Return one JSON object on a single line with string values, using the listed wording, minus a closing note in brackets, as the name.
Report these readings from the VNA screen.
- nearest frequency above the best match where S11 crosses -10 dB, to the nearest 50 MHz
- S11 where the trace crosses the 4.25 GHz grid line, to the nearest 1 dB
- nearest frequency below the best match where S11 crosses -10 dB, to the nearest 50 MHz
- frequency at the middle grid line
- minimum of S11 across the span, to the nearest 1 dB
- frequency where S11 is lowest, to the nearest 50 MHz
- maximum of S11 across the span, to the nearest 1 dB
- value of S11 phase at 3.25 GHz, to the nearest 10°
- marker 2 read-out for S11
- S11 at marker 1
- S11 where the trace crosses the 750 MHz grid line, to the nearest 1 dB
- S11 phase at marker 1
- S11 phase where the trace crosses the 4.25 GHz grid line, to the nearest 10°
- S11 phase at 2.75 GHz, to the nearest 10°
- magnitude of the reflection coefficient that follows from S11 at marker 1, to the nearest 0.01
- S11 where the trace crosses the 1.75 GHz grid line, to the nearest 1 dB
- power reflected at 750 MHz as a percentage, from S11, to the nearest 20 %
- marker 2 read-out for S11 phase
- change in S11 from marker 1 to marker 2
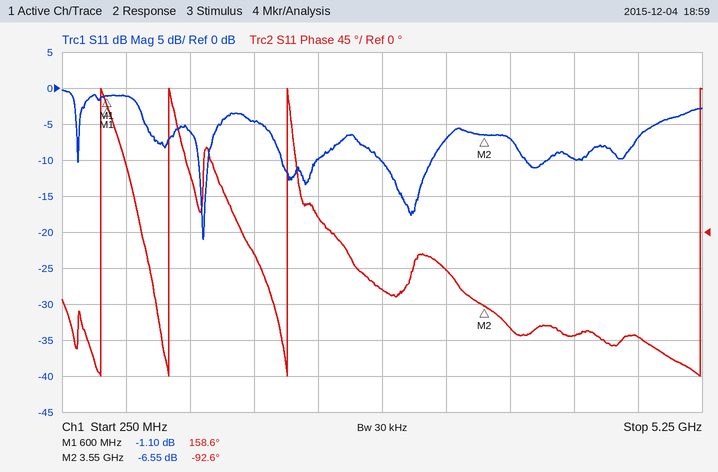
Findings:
{"nearest frequency above the best match where S11 crosses -10 dB, to the nearest 50 MHz": "1.40 GHz", "S11 where the trace crosses the 4.25 GHz grid line, to the nearest 1 dB": "-10 dB", "nearest frequency below the best match where S11 crosses -10 dB, to the nearest 50 MHz": "1.30 GHz", "frequency at the middle grid line": "2.75 GHz", "minimum of S11 across the span, to the nearest 1 dB": "-21 dB", "frequency where S11 is lowest, to the nearest 50 MHz": "1.35 GHz", "maximum of S11 across the span, to the nearest 1 dB": "0 dB", "value of S11 phase at 3.25 GHz, to the nearest 10°": "-50°", "marker 2 read-out for S11": "-6.55 dB", "S11 at marker 1": "-1.10 dB", "S11 where the trace crosses the 750 MHz grid line, to the nearest 1 dB": "-1 dB", "S11 phase at marker 1": "158.6°", "S11 phase where the trace crosses the 4.25 GHz grid line, to the nearest 10°": "-130°", "S11 phase at 2.75 GHz, to the nearest 10°": "-70°", "magnitude of the reflection coefficient that follows from S11 at marker 1, to the nearest 0.01": "0.88", "S11 where the trace crosses the 1.75 GHz grid line, to the nearest 1 dB": "-5 dB", "power reflected at 750 MHz as a percentage, from S11, to the nearest 20 %": "80 %", "marker 2 read-out for S11 phase": "-92.6°", "change in S11 from marker 1 to marker 2": "-5.45 dB"}
